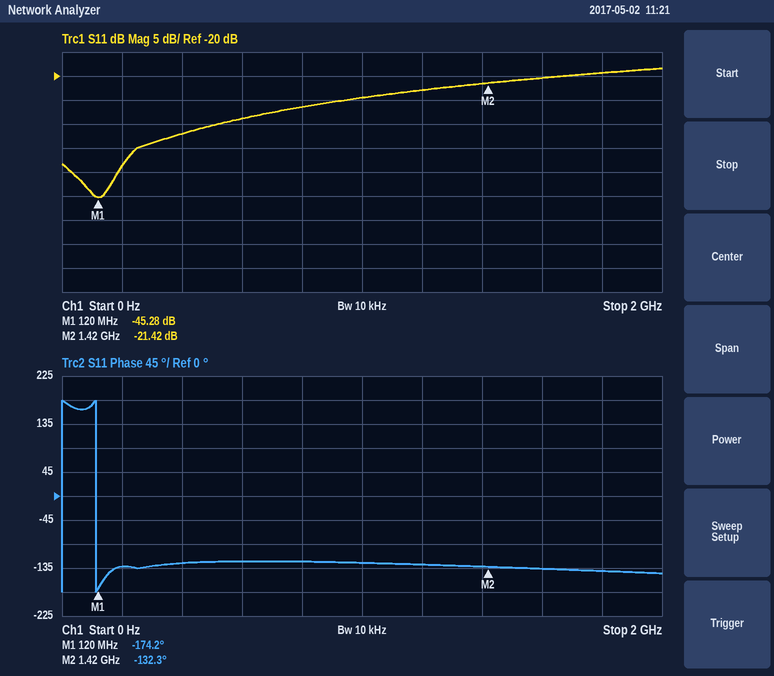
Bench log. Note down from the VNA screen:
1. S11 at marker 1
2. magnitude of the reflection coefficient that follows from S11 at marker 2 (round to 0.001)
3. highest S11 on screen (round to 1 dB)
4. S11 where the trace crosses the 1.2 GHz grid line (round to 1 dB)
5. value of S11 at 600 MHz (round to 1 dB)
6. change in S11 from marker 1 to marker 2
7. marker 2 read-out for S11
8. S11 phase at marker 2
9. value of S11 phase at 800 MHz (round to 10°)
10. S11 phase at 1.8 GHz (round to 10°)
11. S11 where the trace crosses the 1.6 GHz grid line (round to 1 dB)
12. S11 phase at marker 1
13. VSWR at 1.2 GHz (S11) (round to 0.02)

-45.28 dB
0.085
-18 dB
-23 dB
-29 dB
23.86 dB
-21.42 dB
-132.3°
-120°
-140°
-20 dB
-174.2°
1.16
